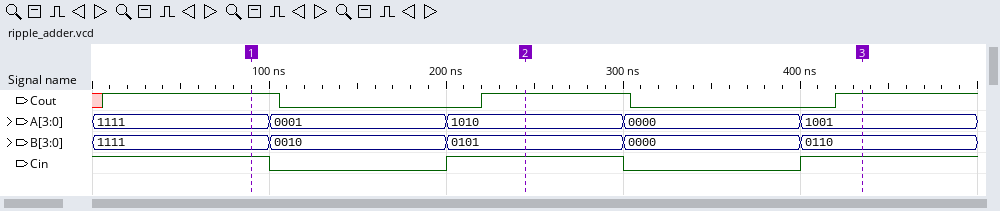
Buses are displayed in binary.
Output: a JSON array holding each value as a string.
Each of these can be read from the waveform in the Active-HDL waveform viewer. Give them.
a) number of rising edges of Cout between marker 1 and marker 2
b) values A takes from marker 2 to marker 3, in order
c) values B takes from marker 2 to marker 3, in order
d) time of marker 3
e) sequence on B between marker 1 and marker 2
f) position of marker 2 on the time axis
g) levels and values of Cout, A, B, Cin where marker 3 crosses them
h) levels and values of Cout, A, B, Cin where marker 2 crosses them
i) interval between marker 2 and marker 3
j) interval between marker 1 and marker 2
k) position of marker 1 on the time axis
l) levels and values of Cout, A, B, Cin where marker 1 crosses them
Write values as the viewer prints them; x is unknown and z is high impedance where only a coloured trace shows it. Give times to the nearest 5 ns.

["1", "1010, 0000, 1001", "0101, 0000, 0110", "435 ns", "1111, 0010, 0101", "245 ns", "Cout=1, A=1001, B=0110, Cin=1", "Cout=1, A=1010, B=0101, Cin=1", "190 ns", "155 ns", "90 ns", "Cout=1, A=1111, B=1111, Cin=1"]
